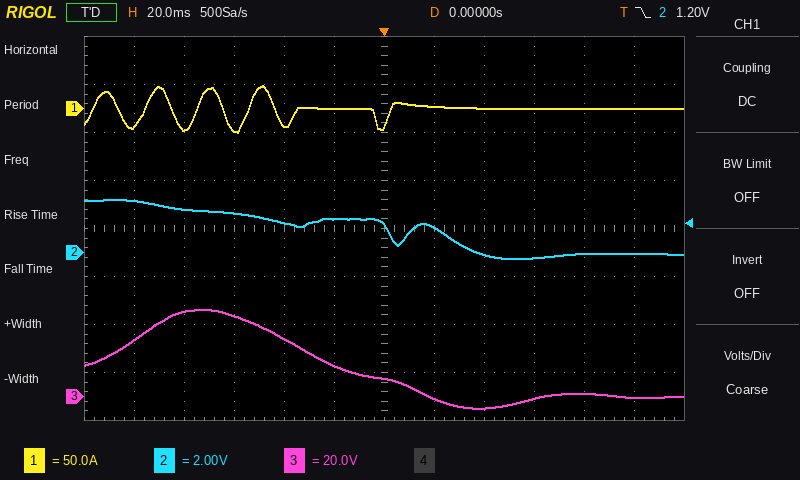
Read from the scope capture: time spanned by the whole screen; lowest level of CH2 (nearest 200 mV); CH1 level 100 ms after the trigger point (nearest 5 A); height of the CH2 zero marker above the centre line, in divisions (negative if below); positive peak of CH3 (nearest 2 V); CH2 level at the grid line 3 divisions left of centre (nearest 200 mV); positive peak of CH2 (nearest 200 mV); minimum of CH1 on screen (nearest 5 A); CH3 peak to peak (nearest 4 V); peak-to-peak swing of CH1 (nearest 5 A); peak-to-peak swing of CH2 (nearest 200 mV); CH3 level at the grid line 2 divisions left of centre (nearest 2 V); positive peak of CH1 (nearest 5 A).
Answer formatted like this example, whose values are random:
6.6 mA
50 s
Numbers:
240 ms
-200 mV
0 A
-0.5 div
36 V
1.6 V
2.2 V
-25 A
40 V
50 A
2.4 V
24 V
25 A
